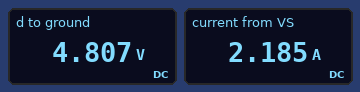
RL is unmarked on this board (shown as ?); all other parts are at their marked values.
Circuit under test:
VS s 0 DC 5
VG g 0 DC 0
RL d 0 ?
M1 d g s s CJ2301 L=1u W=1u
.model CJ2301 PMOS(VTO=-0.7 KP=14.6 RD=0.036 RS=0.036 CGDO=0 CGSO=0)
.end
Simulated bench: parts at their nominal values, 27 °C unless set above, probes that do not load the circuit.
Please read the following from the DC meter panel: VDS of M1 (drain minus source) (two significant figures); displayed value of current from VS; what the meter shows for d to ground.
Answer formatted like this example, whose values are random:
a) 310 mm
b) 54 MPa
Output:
a) -190 mV
b) 2.185 A
c) 4.807 V
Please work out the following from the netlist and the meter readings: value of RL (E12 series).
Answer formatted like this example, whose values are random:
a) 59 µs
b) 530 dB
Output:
a) 2.2 Ω
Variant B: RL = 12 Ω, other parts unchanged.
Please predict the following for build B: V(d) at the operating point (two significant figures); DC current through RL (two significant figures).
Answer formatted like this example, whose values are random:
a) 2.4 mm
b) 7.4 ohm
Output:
a) 5.0 V
b) 410 mA
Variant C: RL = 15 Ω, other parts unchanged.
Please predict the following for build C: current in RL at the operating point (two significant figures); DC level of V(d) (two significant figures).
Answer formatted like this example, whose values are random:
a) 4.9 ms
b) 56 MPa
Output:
a) 330 mA
b) 5.0 V
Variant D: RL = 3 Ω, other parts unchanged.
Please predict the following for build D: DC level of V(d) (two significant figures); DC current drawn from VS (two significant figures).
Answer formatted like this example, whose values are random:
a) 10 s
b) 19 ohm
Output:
a) 4.9 V
b) 1.6 A
